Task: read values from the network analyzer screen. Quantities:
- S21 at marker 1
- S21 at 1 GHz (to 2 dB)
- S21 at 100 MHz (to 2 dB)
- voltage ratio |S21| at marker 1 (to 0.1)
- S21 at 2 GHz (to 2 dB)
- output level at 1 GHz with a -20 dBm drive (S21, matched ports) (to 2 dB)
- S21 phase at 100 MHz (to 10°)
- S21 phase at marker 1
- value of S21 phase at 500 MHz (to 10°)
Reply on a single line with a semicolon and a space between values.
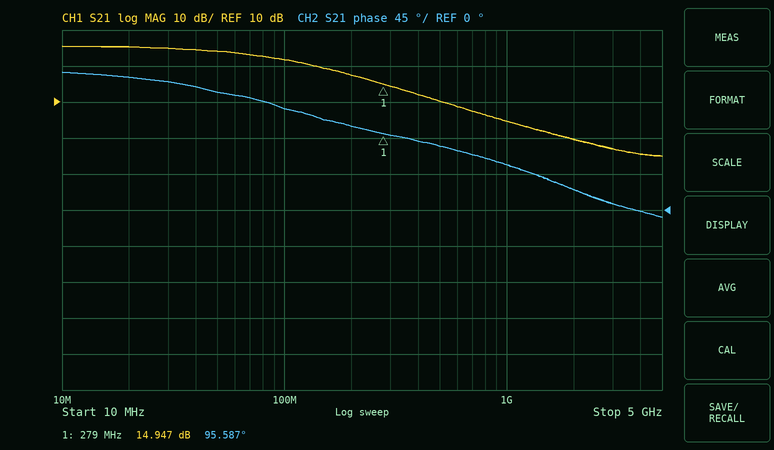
14.947 dB; 4 dB; 22 dB; 5.6; 0 dB; -16 dBm; 130°; 95.587°; 80°
